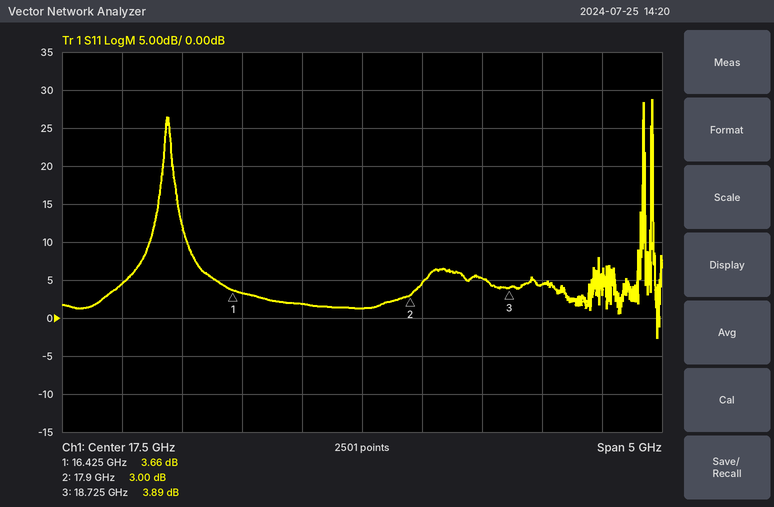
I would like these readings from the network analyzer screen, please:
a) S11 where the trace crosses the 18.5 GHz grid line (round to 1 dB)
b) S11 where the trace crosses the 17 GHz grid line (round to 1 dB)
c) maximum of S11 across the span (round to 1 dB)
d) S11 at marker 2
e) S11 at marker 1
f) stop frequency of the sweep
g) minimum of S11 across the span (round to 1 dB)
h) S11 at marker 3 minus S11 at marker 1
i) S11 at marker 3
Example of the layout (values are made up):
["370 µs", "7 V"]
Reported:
["5 dB", "2 dB", "29 dB", "3.00 dB", "3.66 dB", "20 GHz", "-3 dB", "0.23 dB", "3.89 dB"]
